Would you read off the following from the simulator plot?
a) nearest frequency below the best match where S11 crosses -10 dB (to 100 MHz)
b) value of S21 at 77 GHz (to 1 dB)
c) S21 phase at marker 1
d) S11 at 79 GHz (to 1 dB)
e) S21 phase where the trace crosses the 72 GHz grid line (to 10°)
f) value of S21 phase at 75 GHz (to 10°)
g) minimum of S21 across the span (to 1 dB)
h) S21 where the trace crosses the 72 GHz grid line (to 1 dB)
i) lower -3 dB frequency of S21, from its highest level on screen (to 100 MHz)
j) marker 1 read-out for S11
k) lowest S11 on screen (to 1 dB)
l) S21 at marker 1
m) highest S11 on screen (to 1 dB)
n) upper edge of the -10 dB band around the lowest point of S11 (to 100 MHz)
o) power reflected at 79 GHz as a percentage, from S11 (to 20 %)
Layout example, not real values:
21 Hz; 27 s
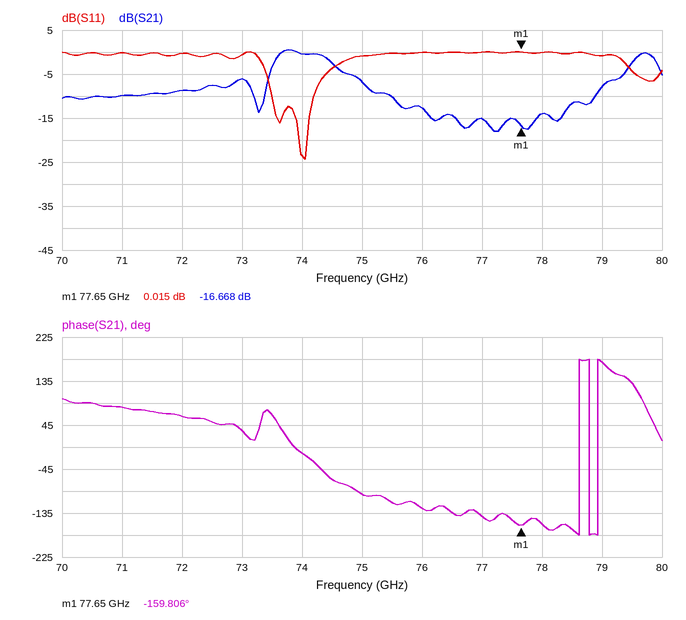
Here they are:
73.5 GHz; -15 dB; -159.806°; -1 dB; 60°; -100°; -18 dB; -9 dB; 73.5 GHz; 0.015 dB; -24 dB; -16.668 dB; 0 dB; 74.2 GHz; 80 %
